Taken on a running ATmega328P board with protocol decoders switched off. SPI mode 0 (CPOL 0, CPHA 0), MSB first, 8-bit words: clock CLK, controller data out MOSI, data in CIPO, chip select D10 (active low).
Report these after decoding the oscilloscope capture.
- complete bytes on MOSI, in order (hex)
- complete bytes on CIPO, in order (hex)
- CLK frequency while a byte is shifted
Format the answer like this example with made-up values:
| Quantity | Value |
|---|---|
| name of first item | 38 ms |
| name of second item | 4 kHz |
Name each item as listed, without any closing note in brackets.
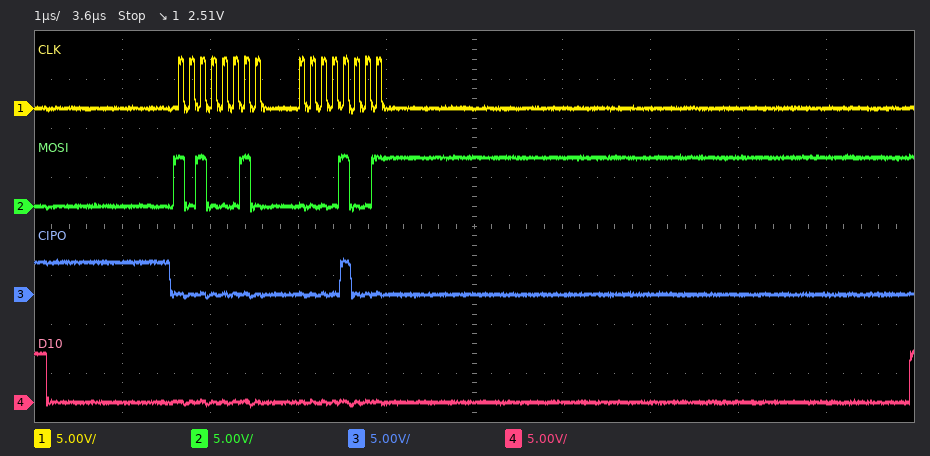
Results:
| Quantity | Value |
|---|---|
| complete bytes on MOSI, in order | A2 09 |
| complete bytes on CIPO, in order | 00 08 |
| CLK frequency while a byte is shifted | 8 MHz |
